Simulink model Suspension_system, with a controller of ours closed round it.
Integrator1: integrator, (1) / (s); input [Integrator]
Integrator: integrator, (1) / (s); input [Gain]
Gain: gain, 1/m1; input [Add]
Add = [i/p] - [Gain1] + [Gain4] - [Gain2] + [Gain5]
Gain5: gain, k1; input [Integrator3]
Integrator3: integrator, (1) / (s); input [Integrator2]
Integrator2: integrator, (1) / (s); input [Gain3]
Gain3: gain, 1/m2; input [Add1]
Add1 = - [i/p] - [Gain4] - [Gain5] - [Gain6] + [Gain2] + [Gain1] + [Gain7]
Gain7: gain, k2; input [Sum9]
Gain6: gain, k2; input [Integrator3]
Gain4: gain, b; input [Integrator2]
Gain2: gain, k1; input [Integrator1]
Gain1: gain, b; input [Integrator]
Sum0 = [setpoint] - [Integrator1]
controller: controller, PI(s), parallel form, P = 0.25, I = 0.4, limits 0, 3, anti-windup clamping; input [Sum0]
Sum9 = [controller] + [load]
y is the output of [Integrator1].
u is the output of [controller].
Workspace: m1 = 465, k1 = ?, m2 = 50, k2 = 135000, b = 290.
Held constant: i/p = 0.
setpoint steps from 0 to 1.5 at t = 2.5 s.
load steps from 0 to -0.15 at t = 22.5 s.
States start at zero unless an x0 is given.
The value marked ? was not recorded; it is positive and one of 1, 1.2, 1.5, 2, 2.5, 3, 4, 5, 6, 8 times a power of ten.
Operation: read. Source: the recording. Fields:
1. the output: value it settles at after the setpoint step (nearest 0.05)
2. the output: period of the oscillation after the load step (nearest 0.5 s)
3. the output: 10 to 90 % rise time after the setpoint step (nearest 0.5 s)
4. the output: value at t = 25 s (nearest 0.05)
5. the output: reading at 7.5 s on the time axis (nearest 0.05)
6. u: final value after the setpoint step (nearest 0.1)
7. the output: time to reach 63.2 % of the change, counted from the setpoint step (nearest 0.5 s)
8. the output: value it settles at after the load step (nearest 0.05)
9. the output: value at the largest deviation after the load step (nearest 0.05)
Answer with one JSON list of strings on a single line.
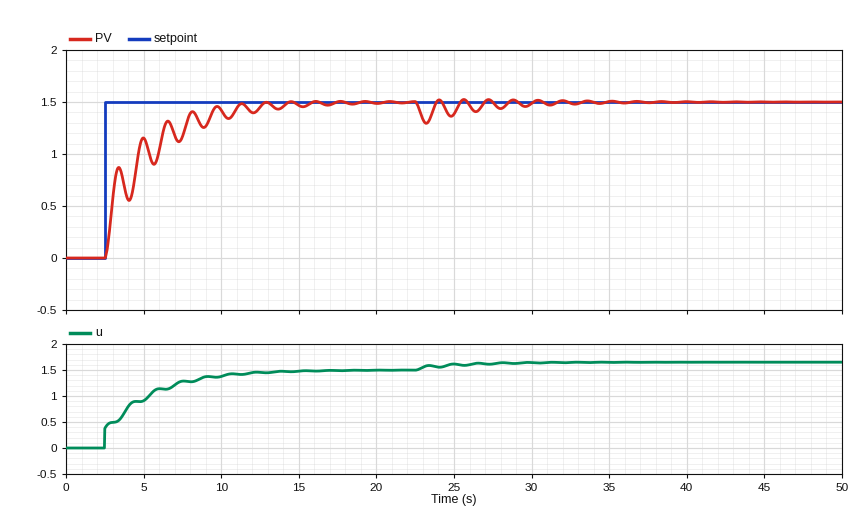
["1.50", "1.5 s", "5.0 s", "1.40", "1.15", "1.5", "2.0 s", "1.50", "1.30"]
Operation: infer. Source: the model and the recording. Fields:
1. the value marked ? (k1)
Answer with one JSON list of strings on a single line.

["6000"]
